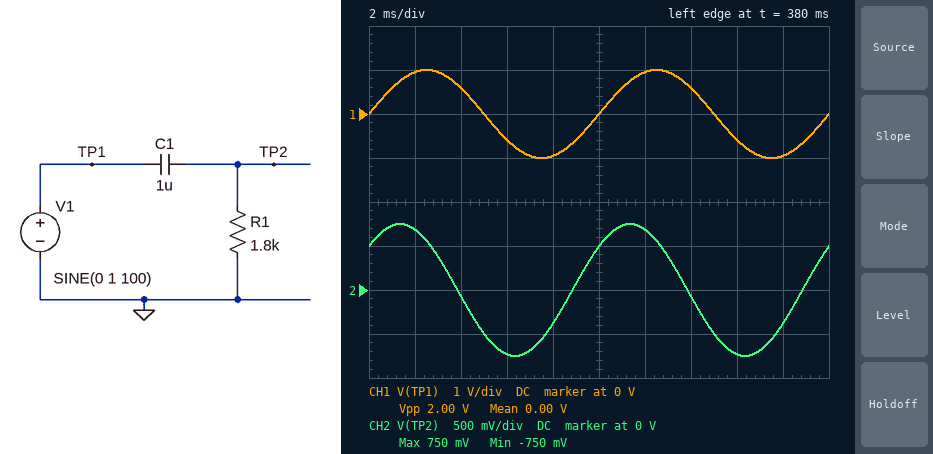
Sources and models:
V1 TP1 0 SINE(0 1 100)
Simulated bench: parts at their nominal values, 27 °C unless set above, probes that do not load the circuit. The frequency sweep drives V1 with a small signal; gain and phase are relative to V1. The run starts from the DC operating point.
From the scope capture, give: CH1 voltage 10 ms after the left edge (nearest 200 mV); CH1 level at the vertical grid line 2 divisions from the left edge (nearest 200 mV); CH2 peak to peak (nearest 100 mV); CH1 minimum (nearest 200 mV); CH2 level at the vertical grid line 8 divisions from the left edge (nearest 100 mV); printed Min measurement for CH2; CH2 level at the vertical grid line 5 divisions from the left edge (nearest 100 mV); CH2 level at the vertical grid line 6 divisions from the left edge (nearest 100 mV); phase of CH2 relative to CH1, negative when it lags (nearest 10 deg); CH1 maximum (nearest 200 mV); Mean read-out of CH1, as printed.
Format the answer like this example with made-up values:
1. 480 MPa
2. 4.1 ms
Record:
1. 0 V
2. 600 mV
3. 1.5 V
4. -1.0 V
5. -700 mV
6. -750 mV
7. 500 mV
8. 700 mV
9. 40 deg
10. 1.0 V
11. 0.00 V
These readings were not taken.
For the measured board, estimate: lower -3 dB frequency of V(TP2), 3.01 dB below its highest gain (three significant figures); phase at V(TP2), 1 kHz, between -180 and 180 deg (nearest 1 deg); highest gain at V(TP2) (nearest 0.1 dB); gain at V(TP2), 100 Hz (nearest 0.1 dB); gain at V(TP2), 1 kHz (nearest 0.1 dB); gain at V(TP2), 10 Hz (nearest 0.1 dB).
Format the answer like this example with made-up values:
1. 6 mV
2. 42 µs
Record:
1. 88.4 Hz
2. 5 deg
3. 0 dB
4. -2.5 dB
5. 0 dB
6. -19.0 dB
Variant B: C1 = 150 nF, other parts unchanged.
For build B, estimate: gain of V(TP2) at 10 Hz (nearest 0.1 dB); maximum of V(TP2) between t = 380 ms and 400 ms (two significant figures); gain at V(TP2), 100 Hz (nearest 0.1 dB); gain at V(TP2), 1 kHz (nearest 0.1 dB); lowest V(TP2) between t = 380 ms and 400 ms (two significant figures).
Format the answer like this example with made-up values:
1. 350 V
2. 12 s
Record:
1. -35.4 dB
2. 170 mV
3. -15.5 dB
4. -1.3 dB
5. -170 mV
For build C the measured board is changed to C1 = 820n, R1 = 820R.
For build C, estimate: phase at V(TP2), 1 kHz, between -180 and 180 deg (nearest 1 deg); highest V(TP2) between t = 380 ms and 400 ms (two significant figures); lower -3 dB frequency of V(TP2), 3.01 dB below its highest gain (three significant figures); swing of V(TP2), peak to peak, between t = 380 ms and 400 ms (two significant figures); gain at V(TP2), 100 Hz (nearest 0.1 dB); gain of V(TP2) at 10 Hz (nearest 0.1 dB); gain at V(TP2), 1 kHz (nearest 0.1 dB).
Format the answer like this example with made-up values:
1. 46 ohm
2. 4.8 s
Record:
1. 13 deg
2. 390 mV
3. 237 Hz
4. 780 mV
5. -8.2 dB
6. -27.5 dB
7. -0.2 dB
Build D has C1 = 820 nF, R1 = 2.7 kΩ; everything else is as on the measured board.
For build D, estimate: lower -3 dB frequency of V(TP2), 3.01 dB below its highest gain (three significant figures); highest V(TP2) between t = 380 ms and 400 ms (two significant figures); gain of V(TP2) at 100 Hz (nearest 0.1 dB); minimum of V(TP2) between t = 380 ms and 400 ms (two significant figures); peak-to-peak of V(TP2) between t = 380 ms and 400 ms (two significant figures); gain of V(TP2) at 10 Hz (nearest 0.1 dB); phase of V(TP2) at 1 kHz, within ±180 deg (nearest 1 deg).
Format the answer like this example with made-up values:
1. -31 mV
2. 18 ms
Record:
1. 71.9 Hz
2. 810 mV
3. -1.8 dB
4. -810 mV
5. 1.6 V
6. -17.2 dB
7. 4 deg
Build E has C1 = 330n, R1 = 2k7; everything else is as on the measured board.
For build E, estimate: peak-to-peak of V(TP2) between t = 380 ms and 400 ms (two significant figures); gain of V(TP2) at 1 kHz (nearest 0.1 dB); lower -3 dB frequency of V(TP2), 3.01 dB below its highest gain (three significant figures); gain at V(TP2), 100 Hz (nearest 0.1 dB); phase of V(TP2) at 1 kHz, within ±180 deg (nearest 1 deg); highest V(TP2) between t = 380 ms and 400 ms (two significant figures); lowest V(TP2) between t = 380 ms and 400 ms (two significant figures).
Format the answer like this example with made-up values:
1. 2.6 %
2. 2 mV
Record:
1. 980 mV
2. -0.1 dB
3. 179 Hz
4. -6.2 dB
5. 10 deg
6. 490 mV
7. -490 mV
